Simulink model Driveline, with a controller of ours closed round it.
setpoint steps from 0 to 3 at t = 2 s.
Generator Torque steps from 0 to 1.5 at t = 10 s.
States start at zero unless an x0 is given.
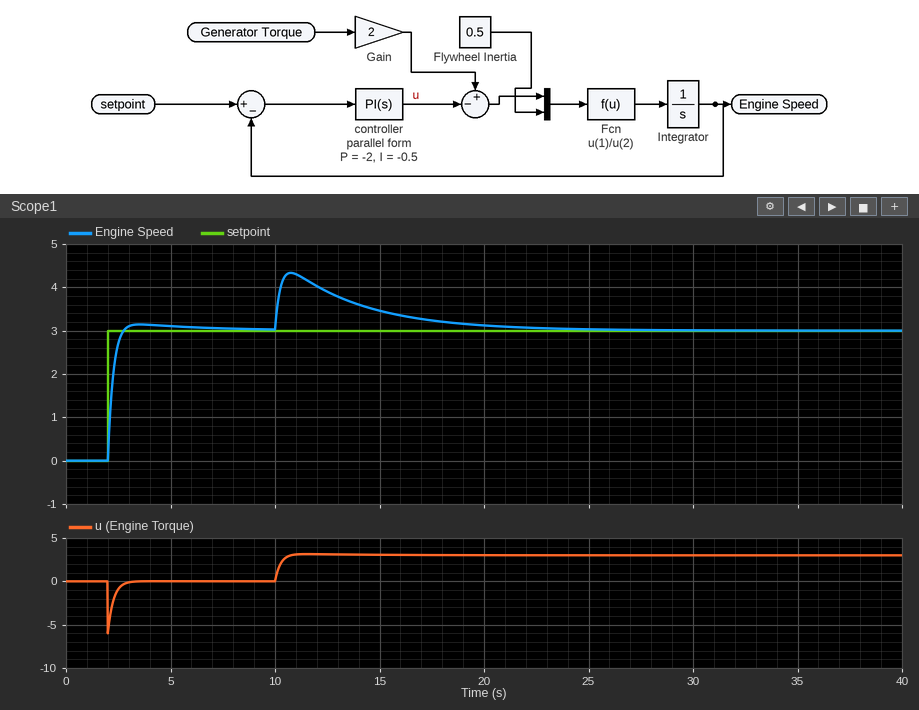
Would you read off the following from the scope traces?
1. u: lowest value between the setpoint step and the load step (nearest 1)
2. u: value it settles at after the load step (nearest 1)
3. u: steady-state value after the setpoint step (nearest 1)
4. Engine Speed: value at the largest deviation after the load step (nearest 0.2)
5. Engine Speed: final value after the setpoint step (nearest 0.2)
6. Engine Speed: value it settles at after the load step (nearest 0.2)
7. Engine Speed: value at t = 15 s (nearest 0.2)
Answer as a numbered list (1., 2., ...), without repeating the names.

1. -6
2. 3
3. 0
4. 4.4
5. 3.0
6. 3.0
7. 3.4
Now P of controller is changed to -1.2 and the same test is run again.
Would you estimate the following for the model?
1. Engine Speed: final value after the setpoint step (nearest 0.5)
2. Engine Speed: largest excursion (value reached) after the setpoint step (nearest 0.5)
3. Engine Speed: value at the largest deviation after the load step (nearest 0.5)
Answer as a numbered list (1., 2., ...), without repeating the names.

1. 3.0
2. 3.5
3. 5.0
